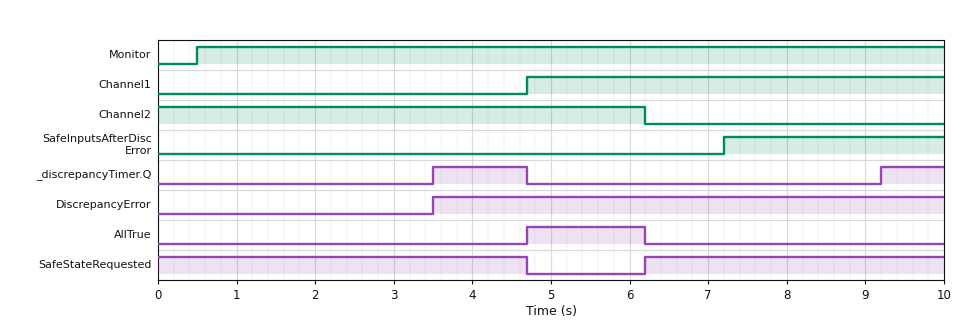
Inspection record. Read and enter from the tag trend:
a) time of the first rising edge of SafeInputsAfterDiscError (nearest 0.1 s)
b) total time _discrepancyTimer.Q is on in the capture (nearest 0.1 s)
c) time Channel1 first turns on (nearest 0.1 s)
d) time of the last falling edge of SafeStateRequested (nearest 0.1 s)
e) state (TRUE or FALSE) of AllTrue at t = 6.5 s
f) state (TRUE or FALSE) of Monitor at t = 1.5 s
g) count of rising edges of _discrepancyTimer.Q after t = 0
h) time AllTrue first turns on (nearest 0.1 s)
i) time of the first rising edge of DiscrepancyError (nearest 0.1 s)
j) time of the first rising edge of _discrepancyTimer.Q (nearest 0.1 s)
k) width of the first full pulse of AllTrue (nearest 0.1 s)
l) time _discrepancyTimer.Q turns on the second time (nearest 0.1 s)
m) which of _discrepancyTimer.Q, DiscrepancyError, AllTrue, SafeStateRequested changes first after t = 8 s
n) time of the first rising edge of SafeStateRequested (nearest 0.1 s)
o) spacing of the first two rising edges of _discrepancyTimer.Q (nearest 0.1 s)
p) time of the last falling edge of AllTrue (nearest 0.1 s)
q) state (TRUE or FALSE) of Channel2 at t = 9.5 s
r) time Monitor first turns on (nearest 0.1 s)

7.2 s
2.0 s
4.7 s
4.7 s
FALSE
TRUE
2
4.7 s
3.5 s
3.5 s
1.5 s
9.2 s
_discrepancyTimer.Q
6.2 s
5.7 s
6.2 s
FALSE
0.5 s
